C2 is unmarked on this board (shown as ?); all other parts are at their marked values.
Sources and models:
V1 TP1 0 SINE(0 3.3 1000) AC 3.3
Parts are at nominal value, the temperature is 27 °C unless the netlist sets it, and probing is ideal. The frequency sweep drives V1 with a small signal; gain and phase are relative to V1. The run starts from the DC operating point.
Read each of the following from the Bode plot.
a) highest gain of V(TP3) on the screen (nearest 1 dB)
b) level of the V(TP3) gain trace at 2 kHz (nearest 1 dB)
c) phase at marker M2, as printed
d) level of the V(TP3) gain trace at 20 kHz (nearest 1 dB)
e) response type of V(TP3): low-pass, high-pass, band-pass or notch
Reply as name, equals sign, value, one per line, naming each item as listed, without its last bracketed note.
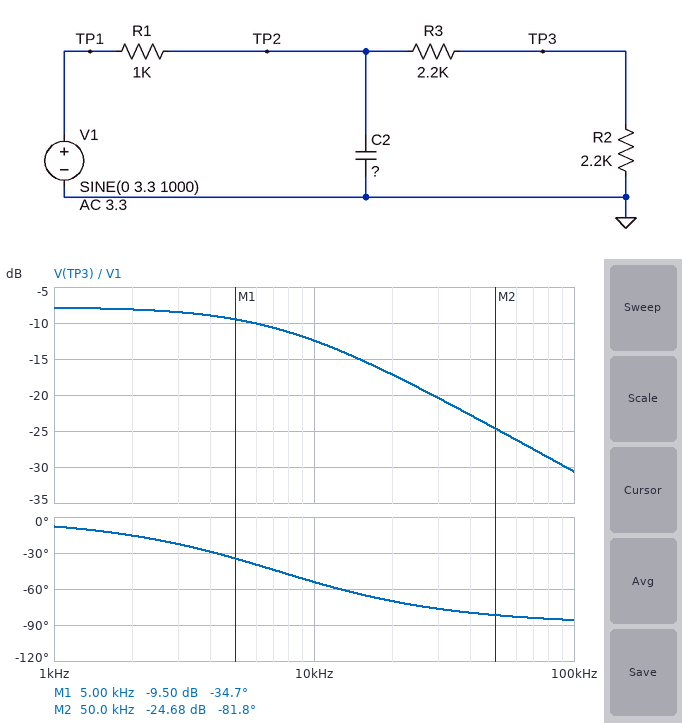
highest gain of V(TP3) on the screen = -8 dB
level of the V(TP3) gain trace at 2 kHz = -8 dB
phase at marker M2, as printed = -81.8 deg
level of the V(TP3) gain trace at 20 kHz = -17 dB
response type of V(TP3): low-pass, high-pass, band-pass or notch = low-pass
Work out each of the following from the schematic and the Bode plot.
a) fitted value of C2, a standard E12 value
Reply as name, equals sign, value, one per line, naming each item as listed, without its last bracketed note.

fitted value of C2, a standard E12 value = 27 nF
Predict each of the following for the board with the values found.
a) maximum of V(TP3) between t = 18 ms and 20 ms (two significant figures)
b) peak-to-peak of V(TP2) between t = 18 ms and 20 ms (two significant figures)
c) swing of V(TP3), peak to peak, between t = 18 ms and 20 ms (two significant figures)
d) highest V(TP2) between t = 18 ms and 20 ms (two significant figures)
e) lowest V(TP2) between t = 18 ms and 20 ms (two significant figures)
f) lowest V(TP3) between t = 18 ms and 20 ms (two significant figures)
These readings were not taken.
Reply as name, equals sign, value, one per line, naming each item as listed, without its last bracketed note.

maximum of V(TP3) between t = 18 ms and 20 ms = 1.3 V
peak-to-peak of V(TP2) between t = 18 ms and 20 ms = 5.3 V
swing of V(TP3), peak to peak, between t = 18 ms and 20 ms = 2.7 V
highest V(TP2) between t = 18 ms and 20 ms = 2.7 V
lowest V(TP2) between t = 18 ms and 20 ms = -2.7 V
lowest V(TP3) between t = 18 ms and 20 ms = -1.3 V
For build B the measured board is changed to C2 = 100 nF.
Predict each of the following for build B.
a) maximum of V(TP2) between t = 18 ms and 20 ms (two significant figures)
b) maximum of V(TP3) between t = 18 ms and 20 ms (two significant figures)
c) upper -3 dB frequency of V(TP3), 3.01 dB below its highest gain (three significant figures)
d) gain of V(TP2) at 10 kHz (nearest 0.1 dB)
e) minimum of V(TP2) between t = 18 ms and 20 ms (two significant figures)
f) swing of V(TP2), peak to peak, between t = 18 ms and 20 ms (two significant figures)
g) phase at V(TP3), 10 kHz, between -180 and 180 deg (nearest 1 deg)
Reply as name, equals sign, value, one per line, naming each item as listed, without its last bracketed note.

maximum of V(TP2) between t = 18 ms and 20 ms = 2.4 V
maximum of V(TP3) between t = 18 ms and 20 ms = 1.2 V
upper -3 dB frequency of V(TP3), 3.01 dB below its highest gain = 1.95 kHz
gain of V(TP2) at 10 kHz = -16.1 dB
minimum of V(TP2) between t = 18 ms and 20 ms = -2.4 V
swing of V(TP2), peak to peak, between t = 18 ms and 20 ms = 4.8 V
phase at V(TP3), 10 kHz, between -180 and 180 deg = -79 deg
